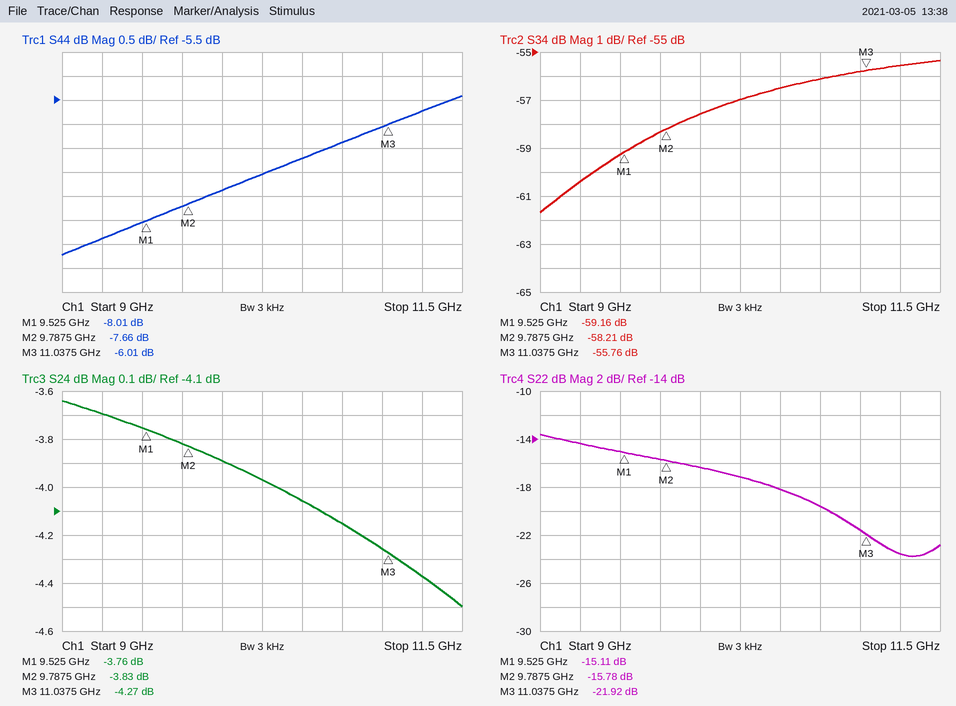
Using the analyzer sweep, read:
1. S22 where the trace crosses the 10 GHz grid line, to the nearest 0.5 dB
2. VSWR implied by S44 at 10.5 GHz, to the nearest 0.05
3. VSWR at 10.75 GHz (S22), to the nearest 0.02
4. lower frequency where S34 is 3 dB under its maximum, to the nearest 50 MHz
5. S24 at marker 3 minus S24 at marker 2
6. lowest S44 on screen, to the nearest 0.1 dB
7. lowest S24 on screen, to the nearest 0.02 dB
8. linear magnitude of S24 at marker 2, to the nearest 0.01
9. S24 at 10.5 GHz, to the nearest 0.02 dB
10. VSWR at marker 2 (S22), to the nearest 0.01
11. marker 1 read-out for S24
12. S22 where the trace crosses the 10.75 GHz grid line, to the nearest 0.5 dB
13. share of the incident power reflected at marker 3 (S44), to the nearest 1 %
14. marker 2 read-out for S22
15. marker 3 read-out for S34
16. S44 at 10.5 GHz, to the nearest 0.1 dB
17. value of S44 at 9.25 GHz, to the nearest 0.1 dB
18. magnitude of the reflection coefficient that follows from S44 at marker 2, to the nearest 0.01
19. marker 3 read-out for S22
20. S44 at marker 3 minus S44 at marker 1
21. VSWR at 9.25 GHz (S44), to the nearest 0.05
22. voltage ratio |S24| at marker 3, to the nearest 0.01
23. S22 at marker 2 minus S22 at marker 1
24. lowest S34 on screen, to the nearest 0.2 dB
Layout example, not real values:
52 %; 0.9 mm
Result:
-16.5 dB; 2.70; 1.24; 9.75 GHz; -0.44 dB; -8.7 dB; -4.50 dB; 0.64; -4.06 dB; 1.39; -3.76 dB; -19.5 dB; 25 %; -15.78 dB; -55.76 dB; -6.7 dB; -8.4 dB; 0.41; -21.92 dB; 2.00 dB; 2.25; 0.61; -0.67 dB; -61.6 dB
